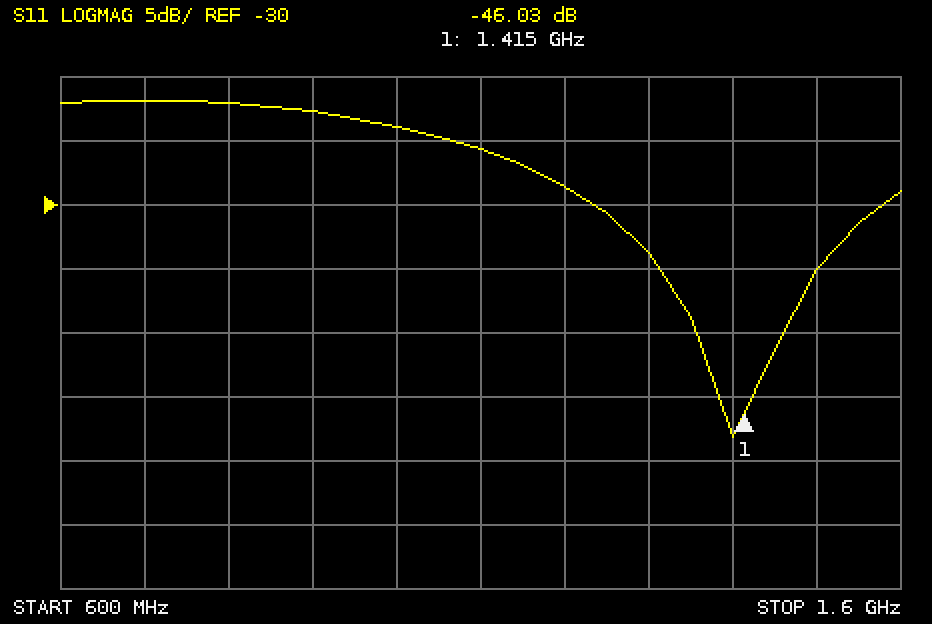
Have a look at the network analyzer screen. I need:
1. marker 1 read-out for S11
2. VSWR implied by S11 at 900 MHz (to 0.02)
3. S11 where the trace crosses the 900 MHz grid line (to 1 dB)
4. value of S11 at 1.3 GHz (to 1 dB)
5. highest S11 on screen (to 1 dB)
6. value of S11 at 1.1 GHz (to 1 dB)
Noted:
-46.03 dB
1.16
-23 dB
-34 dB
-22 dB
-26 dB
